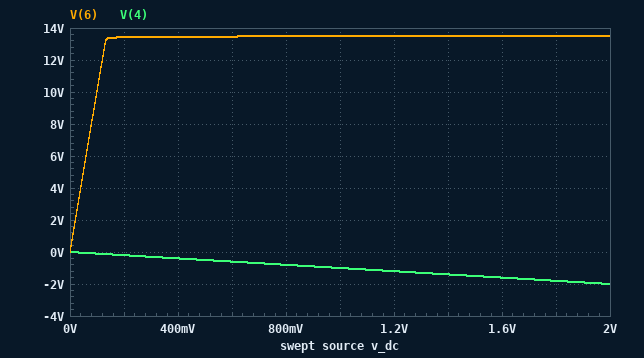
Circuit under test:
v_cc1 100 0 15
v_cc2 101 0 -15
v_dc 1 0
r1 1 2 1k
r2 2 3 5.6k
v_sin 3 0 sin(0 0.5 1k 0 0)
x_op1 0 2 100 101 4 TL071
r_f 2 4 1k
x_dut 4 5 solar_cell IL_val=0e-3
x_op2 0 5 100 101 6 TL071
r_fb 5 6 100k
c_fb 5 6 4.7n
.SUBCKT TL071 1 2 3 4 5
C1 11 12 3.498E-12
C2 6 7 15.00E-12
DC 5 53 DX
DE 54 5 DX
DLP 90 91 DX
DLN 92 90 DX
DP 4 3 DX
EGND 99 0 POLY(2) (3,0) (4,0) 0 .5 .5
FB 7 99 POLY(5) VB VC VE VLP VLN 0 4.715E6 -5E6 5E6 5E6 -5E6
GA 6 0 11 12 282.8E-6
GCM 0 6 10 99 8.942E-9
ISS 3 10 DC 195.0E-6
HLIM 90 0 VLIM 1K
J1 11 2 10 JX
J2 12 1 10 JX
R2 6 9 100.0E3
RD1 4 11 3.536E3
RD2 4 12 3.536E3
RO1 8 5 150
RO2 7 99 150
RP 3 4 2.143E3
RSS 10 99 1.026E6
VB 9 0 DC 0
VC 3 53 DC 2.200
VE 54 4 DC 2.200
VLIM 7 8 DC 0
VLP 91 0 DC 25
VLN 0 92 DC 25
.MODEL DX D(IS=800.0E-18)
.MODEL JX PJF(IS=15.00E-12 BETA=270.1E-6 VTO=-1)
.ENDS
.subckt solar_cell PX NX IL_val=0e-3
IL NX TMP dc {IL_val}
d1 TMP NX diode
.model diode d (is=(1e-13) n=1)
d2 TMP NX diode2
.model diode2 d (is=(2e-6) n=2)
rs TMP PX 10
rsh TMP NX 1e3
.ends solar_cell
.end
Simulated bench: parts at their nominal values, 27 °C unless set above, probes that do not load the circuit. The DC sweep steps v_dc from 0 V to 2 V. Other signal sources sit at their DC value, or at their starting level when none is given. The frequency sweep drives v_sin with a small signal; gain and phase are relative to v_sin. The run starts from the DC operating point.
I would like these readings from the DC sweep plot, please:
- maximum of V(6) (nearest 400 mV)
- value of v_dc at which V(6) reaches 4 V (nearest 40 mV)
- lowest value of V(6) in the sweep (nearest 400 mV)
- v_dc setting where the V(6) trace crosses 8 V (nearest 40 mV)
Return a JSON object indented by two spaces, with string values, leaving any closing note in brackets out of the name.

{
  "maximum of V(6)": "13.6 V",
  "value of v_dc at which V(6) reaches 4 V": "40 mV",
  "lowest value of V(6) in the sweep": "0 V",
  "v_dc setting where the V(6) trace crosses 8 V": "80 mV"
}
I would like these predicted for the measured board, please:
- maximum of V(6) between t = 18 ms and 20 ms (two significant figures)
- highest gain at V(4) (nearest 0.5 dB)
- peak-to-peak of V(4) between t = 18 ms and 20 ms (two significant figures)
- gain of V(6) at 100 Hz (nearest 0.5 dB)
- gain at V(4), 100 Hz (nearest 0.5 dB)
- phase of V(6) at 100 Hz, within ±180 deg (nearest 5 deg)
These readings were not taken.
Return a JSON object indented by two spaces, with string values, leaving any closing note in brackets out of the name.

{
  "maximum of V(6) between t = 18 ms and 20 ms": "2.8 V",
  "highest gain at V(4)": "-15.0 dB",
  "peak-to-peak of V(4) between t = 18 ms and 20 ms": "180 mV",
  "gain of V(6) at 100 Hz": "25.0 dB",
  "gain at V(4), 100 Hz": "-15.0 dB",
  "phase of V(6) at 100 Hz, within ±180 deg": "-15 deg"
}
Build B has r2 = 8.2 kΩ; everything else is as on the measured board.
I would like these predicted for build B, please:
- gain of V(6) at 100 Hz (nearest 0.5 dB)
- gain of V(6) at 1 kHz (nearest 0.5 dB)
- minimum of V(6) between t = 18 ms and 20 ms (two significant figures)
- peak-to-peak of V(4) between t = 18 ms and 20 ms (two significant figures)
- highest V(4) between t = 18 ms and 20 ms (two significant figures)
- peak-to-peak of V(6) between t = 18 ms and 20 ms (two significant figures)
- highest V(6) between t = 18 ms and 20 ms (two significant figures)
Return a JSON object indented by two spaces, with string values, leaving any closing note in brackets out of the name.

{
  "gain of V(6) at 100 Hz": "21.5 dB",
  "gain of V(6) at 1 kHz": "12.0 dB",
  "minimum of V(6) between t = 18 ms and 20 ms": "-2.1 V",
  "peak-to-peak of V(4) between t = 18 ms and 20 ms": "120 mV",
  "highest V(4) between t = 18 ms and 20 ms": "61 mV",
  "peak-to-peak of V(6) between t = 18 ms and 20 ms": "4.0 V",
  "highest V(6) between t = 18 ms and 20 ms": "1.9 V"
}
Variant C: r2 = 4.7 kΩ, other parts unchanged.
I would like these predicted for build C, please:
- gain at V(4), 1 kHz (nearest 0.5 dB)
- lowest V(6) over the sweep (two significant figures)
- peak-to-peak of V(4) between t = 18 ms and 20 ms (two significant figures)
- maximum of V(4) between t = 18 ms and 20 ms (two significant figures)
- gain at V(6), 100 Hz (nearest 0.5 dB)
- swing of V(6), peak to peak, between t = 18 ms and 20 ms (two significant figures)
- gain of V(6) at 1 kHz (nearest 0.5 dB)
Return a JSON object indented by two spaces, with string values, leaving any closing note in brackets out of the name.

{
  "gain at V(4), 1 kHz": "-13.5 dB",
  "lowest V(6) over the sweep": "-1.4 mV",
  "peak-to-peak of V(4) between t = 18 ms and 20 ms": "210 mV",
  "maximum of V(4) between t = 18 ms and 20 ms": "110 mV",
  "gain at V(6), 100 Hz": "26.5 dB",
  "swing of V(6), peak to peak, between t = 18 ms and 20 ms": "7.1 V",
  "gain of V(6) at 1 kHz": "17.0 dB"
}
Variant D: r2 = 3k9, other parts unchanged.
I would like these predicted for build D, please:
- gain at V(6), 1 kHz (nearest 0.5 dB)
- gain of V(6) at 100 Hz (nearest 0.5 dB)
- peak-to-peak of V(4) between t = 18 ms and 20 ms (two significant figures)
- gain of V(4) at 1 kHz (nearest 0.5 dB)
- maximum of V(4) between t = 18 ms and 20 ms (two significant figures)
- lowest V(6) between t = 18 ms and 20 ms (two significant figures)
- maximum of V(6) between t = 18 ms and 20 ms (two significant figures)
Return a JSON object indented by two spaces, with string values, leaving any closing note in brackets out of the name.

{
  "gain at V(6), 1 kHz": "18.5 dB",
  "gain of V(6) at 100 Hz": "28.0 dB",
  "peak-to-peak of V(4) between t = 18 ms and 20 ms": "260 mV",
  "gain of V(4) at 1 kHz": "-12.0 dB",
  "maximum of V(4) between t = 18 ms and 20 ms": "130 mV",
  "lowest V(6) between t = 18 ms and 20 ms": "-4.8 V",
  "maximum of V(6) between t = 18 ms and 20 ms": "3.9 V"
}
